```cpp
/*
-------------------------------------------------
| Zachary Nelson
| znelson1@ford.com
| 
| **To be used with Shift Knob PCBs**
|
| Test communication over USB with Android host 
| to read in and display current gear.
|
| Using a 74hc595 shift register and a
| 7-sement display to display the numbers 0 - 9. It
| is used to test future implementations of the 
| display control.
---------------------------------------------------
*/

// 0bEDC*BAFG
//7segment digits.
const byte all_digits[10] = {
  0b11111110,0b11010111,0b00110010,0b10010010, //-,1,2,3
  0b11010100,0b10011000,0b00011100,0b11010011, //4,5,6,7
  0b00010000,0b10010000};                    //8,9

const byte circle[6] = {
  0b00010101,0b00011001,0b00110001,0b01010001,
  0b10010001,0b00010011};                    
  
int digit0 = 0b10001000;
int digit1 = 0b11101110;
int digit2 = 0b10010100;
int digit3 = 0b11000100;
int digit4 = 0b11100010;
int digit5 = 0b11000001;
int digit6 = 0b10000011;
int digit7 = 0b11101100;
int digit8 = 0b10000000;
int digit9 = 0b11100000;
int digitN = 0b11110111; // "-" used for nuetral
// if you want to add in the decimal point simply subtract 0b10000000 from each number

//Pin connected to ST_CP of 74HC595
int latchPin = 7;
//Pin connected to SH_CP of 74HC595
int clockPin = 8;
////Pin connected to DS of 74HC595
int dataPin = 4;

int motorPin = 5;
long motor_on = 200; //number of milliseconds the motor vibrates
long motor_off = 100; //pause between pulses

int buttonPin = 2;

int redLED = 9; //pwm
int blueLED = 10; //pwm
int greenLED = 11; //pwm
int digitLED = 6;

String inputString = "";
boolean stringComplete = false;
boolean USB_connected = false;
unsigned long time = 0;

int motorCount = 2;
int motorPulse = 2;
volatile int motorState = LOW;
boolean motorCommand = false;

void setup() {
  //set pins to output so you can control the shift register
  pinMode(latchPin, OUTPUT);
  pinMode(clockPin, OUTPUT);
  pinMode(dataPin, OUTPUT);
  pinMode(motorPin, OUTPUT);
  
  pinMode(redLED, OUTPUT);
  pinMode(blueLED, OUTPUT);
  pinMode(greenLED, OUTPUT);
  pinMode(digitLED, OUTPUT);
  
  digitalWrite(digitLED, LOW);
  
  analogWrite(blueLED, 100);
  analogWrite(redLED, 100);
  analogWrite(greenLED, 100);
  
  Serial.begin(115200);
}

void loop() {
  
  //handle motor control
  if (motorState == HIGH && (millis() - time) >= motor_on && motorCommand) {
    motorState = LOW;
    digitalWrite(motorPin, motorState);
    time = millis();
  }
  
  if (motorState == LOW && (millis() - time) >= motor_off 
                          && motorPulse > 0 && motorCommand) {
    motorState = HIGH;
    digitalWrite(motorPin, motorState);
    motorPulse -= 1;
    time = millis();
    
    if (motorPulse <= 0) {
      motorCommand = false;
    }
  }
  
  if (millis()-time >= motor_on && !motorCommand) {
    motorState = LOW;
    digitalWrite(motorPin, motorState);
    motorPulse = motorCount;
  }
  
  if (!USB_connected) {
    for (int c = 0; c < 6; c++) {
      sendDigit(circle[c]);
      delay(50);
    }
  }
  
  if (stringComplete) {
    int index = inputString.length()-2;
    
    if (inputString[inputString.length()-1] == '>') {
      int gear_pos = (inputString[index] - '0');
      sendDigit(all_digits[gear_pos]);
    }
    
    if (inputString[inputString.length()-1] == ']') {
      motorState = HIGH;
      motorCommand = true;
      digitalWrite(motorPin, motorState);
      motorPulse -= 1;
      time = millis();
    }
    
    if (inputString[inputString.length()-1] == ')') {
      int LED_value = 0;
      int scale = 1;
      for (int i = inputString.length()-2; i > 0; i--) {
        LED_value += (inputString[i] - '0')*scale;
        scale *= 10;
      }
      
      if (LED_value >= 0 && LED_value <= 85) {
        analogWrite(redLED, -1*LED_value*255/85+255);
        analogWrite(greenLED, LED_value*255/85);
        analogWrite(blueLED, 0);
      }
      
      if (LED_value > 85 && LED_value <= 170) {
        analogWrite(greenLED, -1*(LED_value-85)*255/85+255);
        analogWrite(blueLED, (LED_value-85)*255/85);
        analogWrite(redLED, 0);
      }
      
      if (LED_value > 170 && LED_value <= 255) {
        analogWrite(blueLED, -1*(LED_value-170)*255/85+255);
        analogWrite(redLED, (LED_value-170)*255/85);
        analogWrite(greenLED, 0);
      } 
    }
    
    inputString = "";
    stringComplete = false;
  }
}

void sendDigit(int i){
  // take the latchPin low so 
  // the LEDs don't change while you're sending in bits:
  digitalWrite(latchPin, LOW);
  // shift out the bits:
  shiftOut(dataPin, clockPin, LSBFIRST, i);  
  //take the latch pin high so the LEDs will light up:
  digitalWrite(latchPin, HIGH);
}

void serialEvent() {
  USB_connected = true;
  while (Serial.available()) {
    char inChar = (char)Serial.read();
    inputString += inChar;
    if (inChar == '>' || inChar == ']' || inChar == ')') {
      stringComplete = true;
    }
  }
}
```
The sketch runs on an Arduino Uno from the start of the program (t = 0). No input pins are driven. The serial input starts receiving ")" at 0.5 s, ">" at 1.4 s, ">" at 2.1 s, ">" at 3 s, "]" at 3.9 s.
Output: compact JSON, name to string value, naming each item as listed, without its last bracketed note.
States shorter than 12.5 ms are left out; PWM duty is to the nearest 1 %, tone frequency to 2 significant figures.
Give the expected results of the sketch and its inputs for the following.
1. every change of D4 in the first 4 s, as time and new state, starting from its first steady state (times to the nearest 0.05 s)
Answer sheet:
{"every change of D4 in the first 4 s, as time and new state, starting from its first steady state": "0 s low; 0.2 s high; 0.25 s low; 0.5 s high; 0.55 s low"}
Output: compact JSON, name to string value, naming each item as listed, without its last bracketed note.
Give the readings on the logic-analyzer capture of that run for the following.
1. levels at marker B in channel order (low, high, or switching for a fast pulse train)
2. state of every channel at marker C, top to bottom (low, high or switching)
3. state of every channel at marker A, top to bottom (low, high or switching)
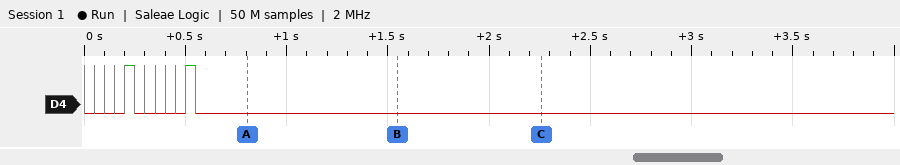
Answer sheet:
{"levels at marker B in channel order": "D4 low", "state of every channel at marker C, top to bottom": "D4 low", "state of every channel at marker A, top to bottom": "D4 low"}
